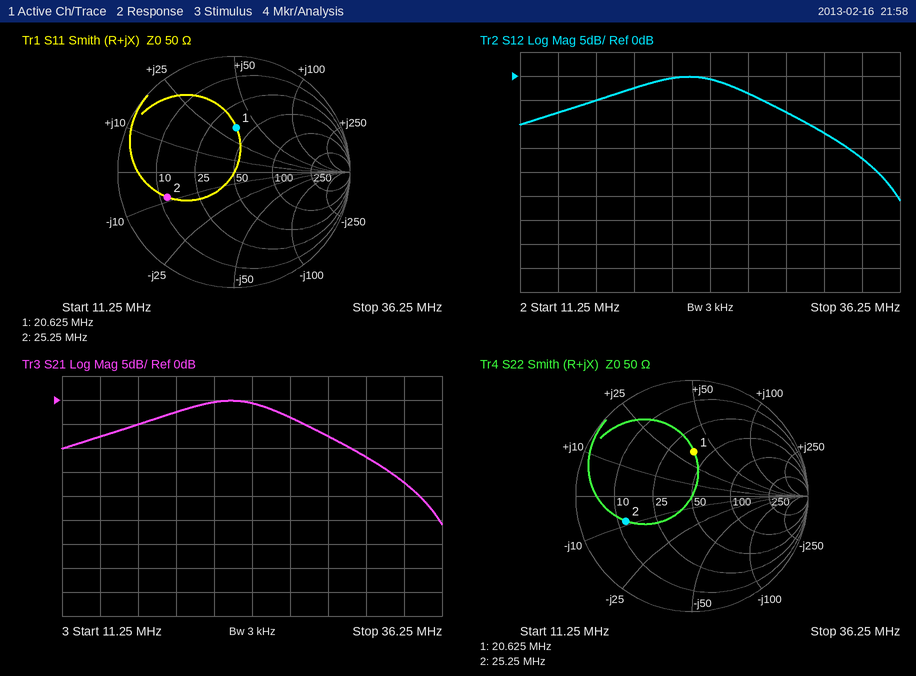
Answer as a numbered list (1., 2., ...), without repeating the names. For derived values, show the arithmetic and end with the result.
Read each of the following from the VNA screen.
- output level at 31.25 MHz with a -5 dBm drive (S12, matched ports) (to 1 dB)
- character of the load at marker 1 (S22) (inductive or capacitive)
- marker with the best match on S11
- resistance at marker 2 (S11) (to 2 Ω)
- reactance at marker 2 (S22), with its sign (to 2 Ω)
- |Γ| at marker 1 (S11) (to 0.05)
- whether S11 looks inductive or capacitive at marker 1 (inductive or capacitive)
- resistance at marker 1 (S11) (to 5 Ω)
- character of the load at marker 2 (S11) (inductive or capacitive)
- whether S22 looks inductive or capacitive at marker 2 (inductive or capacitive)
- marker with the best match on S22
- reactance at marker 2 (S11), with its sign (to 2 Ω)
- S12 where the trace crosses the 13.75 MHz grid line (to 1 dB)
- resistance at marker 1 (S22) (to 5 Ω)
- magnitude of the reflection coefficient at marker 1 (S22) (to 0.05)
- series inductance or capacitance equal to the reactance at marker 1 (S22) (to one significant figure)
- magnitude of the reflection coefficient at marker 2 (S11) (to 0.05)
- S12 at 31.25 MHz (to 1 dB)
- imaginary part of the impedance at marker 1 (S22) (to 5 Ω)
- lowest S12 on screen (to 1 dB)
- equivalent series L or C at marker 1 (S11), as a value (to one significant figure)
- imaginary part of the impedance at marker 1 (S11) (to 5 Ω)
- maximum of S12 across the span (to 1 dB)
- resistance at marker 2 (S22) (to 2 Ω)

1. -5 dBm + (-12 dB) = -17 dBm
2. inductive
3. marker 1
4. 12 Ω
5. -8 Ω
6. 0.40
7. inductive
8. 40 Ω
9. capacitive
10. capacitive
11. marker 1
12. -8 Ω
13. -8 dB
14. 40 Ω
15. 0.40
16. L = 35 Ω/(2π × 20.625 MHz) ≈ 270 nH, so 300 nH to one significant figure
17. 0.60
18. -12 dB
19. +35 Ω
20. -26 dB
21. L = 35 Ω/(2π × 20.625 MHz) ≈ 270 nH, so 300 nH to one significant figure
22. +35 Ω
23. 0 dB
24. 12 Ω
